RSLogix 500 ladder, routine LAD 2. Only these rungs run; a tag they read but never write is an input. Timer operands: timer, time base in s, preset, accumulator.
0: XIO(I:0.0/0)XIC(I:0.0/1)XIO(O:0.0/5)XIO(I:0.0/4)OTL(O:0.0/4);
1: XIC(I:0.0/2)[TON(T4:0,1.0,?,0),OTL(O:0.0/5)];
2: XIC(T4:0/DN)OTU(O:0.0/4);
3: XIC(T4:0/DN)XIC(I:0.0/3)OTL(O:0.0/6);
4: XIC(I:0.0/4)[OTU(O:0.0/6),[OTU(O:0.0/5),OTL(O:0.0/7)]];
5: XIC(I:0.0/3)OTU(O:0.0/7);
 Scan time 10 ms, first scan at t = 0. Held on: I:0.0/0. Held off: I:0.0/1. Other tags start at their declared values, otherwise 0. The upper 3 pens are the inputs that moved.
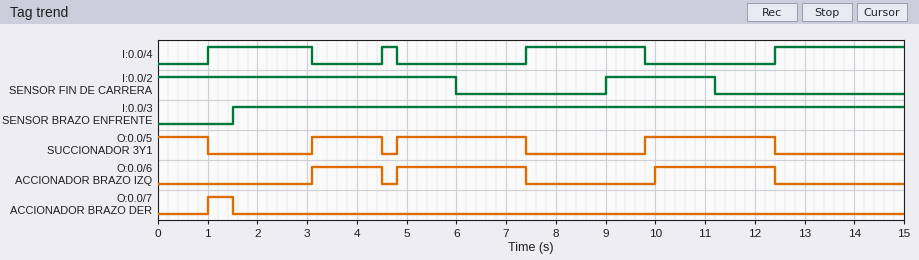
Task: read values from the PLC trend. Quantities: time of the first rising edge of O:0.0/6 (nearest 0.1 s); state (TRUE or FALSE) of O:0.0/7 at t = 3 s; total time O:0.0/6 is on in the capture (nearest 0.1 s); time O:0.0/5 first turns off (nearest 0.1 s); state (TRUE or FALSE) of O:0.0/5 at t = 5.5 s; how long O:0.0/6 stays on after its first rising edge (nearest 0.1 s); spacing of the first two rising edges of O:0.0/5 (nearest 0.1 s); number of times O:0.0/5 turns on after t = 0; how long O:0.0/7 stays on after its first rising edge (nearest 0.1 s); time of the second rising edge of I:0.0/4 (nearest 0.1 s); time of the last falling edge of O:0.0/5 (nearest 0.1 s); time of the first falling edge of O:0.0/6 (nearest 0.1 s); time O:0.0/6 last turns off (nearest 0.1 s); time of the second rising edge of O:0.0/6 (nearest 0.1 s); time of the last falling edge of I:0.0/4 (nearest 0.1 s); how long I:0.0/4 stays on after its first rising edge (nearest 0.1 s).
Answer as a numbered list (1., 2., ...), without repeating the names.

1. 3.1 s
2. FALSE
3. 6.4 s
4. 1.0 s
5. TRUE
6. 1.4 s
7. 1.7 s
8. 3
9. 0.5 s
10. 4.5 s
11. 12.4 s
12. 4.5 s
13. 12.4 s
14. 4.8 s
15. 9.8 s
16. 2.1 s
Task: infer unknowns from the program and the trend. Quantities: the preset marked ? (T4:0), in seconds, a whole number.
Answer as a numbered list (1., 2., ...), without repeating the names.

1. 1 s
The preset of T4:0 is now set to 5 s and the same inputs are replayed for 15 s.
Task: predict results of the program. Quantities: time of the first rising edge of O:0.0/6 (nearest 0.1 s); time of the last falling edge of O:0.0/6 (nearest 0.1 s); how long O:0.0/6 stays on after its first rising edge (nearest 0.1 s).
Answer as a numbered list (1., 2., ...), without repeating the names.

1. 5.0 s
2. 7.4 s
3. 2.4 s
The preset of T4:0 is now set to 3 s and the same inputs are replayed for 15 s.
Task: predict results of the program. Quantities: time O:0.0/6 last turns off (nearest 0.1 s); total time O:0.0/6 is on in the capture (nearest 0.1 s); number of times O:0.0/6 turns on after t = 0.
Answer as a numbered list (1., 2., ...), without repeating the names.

1. 7.4 s
2. 4.0 s
3. 2
